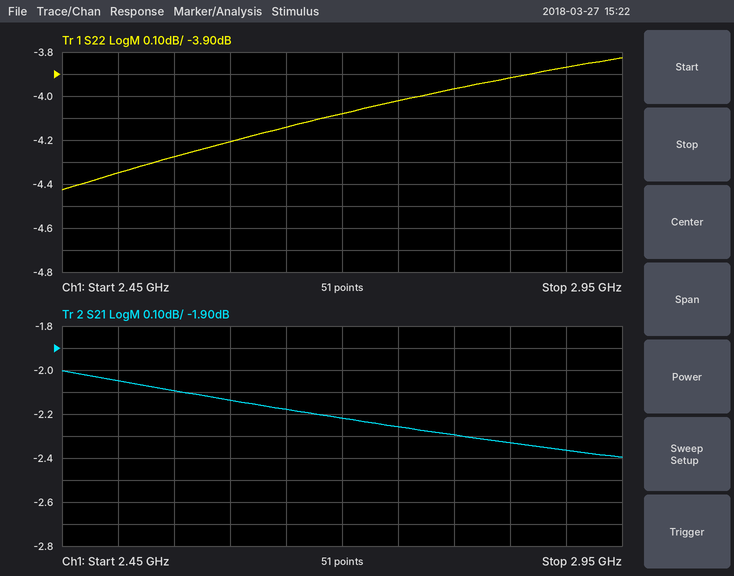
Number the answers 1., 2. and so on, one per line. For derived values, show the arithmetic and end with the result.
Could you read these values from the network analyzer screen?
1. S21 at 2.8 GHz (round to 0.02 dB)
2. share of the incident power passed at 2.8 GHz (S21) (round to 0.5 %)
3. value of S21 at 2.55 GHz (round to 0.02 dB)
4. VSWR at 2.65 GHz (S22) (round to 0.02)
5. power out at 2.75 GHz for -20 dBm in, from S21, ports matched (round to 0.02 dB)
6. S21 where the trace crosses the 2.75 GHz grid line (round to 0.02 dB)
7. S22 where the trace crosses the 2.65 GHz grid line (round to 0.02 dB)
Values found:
1. -2.30 dB
2. 10^(-2.3/10) ≈ 58.9 %, so 59.0 % to the nearest 0.5 %
3. -2.10 dB
4. |Γ| = 10^(-4.14/20) = 0.6209; VSWR = (1 + 0.6209)/(1 − 0.6209) ≈ 4.28
5. -20 dBm + (-2.26 dB) = -22.26 dBm
6. -2.26 dB
7. -4.14 dB
